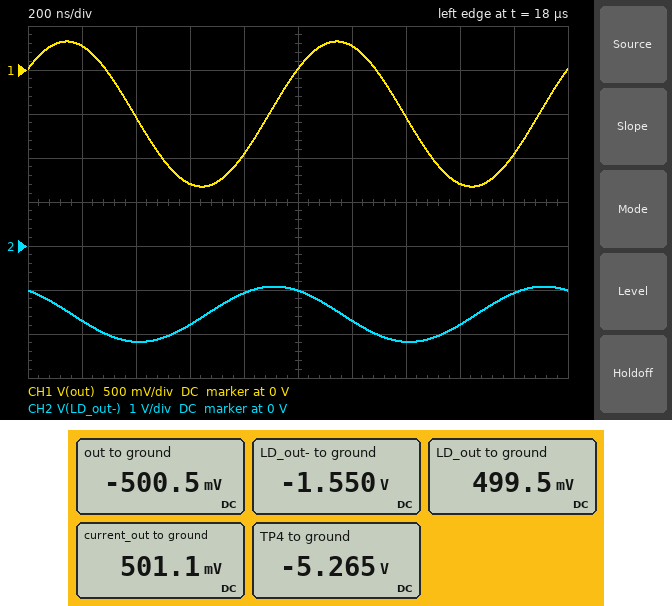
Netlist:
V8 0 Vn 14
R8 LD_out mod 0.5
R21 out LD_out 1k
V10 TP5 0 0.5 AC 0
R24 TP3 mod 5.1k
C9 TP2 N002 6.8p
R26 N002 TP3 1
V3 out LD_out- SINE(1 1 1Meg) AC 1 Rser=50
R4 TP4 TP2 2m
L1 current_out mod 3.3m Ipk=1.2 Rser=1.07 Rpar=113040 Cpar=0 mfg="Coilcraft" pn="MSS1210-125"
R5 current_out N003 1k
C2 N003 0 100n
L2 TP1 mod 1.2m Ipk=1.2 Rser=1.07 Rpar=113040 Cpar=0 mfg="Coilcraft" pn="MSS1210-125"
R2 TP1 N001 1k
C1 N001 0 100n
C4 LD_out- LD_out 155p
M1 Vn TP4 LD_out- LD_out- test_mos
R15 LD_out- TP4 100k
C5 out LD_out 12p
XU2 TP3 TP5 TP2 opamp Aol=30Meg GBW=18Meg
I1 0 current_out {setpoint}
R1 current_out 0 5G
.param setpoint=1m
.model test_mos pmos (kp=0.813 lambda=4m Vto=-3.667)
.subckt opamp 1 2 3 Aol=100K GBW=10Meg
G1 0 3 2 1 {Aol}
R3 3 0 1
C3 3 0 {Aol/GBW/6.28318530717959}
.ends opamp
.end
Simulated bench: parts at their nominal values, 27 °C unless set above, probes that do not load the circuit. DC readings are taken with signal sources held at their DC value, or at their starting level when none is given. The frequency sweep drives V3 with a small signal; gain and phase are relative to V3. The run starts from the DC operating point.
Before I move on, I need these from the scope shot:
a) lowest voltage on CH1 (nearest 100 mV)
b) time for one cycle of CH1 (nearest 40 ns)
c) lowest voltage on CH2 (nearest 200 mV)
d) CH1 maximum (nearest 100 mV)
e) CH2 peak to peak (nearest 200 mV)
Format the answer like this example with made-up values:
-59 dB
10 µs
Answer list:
-1.3 V
1.00 µs
-2.2 V
300 mV
1.2 V
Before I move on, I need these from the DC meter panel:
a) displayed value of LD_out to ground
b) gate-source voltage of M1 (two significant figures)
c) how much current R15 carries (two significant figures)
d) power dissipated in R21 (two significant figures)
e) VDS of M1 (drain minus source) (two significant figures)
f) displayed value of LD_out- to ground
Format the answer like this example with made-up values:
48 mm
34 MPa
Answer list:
499.5 mV
-3.7 V
37 µA
1.0 mW
-12 V
-1.550 V
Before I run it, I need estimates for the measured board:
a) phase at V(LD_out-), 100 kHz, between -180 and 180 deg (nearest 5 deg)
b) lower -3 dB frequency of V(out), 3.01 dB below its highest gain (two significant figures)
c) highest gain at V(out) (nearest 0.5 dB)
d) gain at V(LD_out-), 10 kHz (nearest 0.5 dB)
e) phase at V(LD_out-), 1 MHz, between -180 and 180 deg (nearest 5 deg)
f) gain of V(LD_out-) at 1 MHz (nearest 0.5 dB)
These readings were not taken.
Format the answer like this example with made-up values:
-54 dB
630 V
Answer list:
170 deg
790 kHz
0.5 dB
0 dB
120 deg
-4.0 dB
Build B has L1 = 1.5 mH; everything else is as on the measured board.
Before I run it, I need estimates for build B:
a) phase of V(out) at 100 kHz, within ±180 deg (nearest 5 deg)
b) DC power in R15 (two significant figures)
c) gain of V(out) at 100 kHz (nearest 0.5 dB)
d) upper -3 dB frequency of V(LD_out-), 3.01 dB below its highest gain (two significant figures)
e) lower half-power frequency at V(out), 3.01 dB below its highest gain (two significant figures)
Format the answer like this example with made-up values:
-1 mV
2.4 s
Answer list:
70 deg
140 µW
-16.0 dB
780 kHz
800 kHz
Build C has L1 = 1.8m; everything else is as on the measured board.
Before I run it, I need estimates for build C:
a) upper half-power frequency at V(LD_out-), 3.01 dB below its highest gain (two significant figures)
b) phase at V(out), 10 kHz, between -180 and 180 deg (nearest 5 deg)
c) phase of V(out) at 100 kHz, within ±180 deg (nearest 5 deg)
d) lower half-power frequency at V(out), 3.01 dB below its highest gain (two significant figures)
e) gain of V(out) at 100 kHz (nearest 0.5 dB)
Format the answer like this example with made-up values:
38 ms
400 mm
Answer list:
790 kHz
90 deg
70 deg
800 kHz
-16.0 dB
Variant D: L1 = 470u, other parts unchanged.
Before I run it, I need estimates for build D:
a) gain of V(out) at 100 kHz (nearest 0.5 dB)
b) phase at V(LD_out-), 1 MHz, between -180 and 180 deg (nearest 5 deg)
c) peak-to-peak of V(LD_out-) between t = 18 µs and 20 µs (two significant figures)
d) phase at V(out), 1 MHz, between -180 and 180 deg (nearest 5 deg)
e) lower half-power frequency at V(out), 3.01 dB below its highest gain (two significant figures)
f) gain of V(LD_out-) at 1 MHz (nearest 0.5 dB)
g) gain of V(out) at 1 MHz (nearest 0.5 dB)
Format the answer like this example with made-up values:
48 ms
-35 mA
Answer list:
-15.5 dB
125 deg
1.2 V
35 deg
820 kHz
-4.5 dB
-2.0 dB
